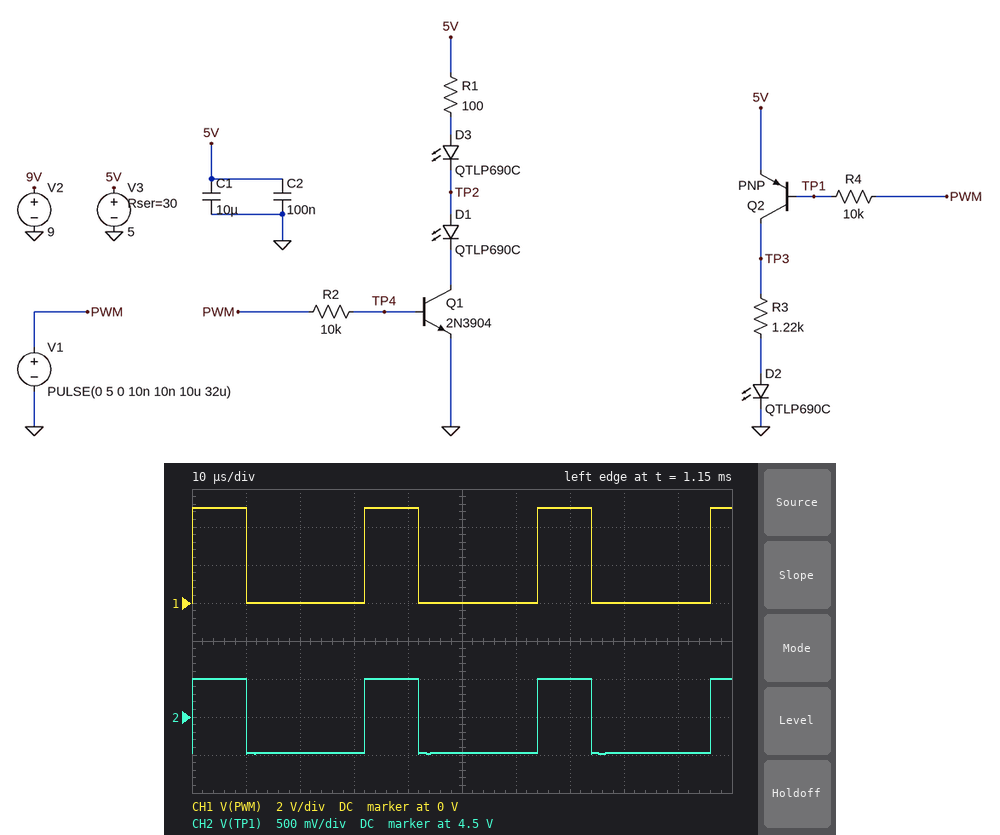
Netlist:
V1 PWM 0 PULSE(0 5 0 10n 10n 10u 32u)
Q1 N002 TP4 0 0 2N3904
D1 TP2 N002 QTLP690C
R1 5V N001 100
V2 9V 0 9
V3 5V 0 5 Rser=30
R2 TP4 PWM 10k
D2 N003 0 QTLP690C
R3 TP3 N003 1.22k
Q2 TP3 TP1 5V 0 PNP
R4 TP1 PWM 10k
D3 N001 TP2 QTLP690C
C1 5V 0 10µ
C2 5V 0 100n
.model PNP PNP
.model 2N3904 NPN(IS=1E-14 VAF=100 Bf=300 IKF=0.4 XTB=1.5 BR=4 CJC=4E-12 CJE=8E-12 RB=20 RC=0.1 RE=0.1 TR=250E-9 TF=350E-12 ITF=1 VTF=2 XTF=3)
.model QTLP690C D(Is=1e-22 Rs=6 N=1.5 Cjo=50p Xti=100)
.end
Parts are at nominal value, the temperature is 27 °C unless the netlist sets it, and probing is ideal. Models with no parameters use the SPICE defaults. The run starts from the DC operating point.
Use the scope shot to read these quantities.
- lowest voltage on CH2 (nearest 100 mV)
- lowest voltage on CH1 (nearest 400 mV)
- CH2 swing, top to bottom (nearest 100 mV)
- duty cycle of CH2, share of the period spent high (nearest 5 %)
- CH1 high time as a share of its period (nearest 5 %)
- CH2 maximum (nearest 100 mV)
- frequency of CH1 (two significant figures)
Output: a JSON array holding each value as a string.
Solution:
["4.0 V", "0 V", "1.0 V", "30 %", "30 %", "5.0 V", "31 kHz"]
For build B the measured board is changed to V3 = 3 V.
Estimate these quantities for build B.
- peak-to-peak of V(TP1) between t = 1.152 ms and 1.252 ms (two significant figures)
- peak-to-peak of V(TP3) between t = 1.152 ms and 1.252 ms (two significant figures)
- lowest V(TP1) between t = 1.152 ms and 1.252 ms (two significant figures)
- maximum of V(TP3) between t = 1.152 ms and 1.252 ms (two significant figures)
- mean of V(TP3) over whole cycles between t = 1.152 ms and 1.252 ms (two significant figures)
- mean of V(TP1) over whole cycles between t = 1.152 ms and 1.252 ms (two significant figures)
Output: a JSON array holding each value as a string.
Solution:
["2.8 V", "1.5 V", "2.2 V", "2.9 V", "2.5 V", "3.1 V"]
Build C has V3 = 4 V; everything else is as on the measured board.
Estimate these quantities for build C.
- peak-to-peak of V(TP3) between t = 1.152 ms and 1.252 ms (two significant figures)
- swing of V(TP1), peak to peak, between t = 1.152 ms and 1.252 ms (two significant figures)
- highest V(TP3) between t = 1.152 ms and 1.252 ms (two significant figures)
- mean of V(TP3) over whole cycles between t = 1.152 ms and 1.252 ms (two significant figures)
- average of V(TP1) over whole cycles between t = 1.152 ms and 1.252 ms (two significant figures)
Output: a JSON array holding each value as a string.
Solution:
["2.5 V", "1.9 V", "3.9 V", "3.1 V", "3.7 V"]
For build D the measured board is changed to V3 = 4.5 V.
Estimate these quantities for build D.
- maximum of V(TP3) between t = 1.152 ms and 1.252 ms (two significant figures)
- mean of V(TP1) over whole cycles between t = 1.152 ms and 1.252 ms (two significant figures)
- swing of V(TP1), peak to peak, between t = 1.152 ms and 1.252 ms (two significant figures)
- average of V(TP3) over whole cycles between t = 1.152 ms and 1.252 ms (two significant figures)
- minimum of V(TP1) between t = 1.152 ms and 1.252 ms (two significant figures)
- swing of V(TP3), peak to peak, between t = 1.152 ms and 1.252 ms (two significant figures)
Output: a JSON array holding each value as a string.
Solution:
["4.3 V", "4.0 V", "1.4 V", "3.4 V", "3.6 V", "2.9 V"]
